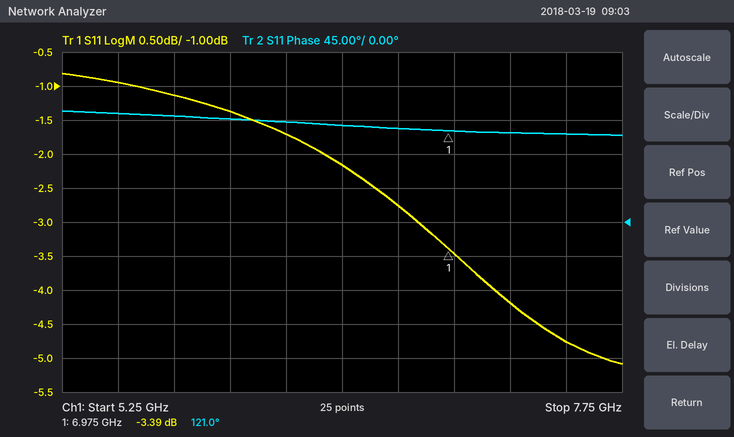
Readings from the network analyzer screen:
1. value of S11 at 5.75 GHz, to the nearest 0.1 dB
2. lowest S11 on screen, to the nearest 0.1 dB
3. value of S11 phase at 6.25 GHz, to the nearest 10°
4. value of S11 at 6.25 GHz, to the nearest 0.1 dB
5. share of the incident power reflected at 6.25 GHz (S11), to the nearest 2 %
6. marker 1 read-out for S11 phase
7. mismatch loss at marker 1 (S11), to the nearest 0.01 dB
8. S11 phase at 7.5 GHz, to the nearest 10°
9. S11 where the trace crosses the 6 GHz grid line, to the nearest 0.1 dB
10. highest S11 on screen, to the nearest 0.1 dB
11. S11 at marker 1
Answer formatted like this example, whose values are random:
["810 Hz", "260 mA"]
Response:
["-1.1 dB", "-5.1 dB", "130°", "-1.7 dB", "68 %", "121.0°", "2.66 dB", "120°", "-1.4 dB", "-0.8 dB", "-3.39 dB"]
